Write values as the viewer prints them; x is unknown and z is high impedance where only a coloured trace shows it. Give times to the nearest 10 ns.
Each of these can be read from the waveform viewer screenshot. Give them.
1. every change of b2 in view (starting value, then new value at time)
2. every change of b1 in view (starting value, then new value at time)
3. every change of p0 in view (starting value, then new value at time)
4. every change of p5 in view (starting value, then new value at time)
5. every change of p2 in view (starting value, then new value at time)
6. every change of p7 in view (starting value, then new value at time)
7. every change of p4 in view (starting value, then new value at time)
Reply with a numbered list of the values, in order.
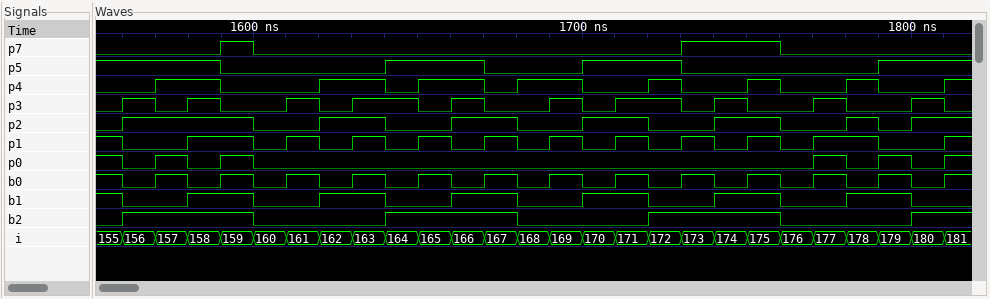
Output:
1. 0, 1 at 1560 ns, 0 at 1600 ns, 1 at 1640 ns, 0 at 1680 ns, 1 at 1720 ns, 0 at 1760 ns, 1 at 1800 ns
2. 1, 0 at 1560 ns, 1 at 1580 ns, 0 at 1600 ns, 1 at 1620 ns, 0 at 1640 ns, 1 at 1660 ns, 0 at 1680 ns, 1 at 1700 ns, 0 at 1720 ns, 1 at 1740 ns, 0 at 1760 ns, 1 at 1780 ns, 0 at 1800 ns
3. 1, 0 at 1560 ns, 1 at 1570 ns, 0 at 1580 ns, 1 at 1590 ns, 0 at 1600 ns, 1 at 1770 ns, 0 at 1780 ns, 1 at 1790 ns, 0 at 1800 ns, 1 at 1810 ns
4. 1, 0 at 1590 ns, 1 at 1640 ns, 0 at 1670 ns, 1 at 1700 ns, 0 at 1730 ns, 1 at 1790 ns
5. 0, 1 at 1560 ns, 0 at 1600 ns, 1 at 1620 ns, 0 at 1640 ns, 1 at 1660 ns, 0 at 1680 ns, 1 at 1700 ns, 0 at 1720 ns, 1 at 1740 ns, 0 at 1760 ns, 1 at 1780 ns, 0 at 1790 ns, 1 at 1800 ns
6. 0, 1 at 1590 ns, 0 at 1600 ns, 1 at 1730 ns, 0 at 1760 ns
7. 0, 1 at 1570 ns, 0 at 1590 ns, 1 at 1620 ns, 0 at 1640 ns, 1 at 1650 ns, 0 at 1670 ns, 1 at 1680 ns, 0 at 1700 ns, 1 at 1720 ns, 0 at 1730 ns, 1 at 1750 ns, 0 at 1760 ns, 1 at 1780 ns, 0 at 1790 ns, 1 at 1810 ns
